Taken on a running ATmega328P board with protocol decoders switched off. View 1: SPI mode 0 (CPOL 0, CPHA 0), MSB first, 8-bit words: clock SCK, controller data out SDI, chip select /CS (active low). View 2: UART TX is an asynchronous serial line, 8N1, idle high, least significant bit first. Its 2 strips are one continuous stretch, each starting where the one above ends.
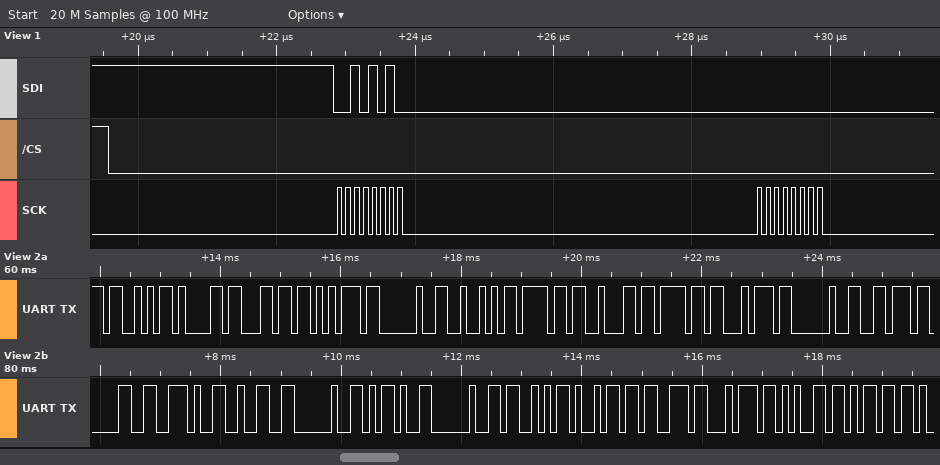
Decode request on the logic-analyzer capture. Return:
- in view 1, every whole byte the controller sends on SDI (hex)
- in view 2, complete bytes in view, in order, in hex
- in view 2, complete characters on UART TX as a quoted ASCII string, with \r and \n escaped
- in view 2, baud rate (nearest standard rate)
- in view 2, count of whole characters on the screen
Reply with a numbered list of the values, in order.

1. 2A 00
2. 53 61 6C 75 20 52 6F 62 6F 74 20 76 30 2E 32 20 2D 20 53 69 73 74 65 6D
3. "Salu Robot v0.2 - Sistem"
4. 9600 baud
5. 24
